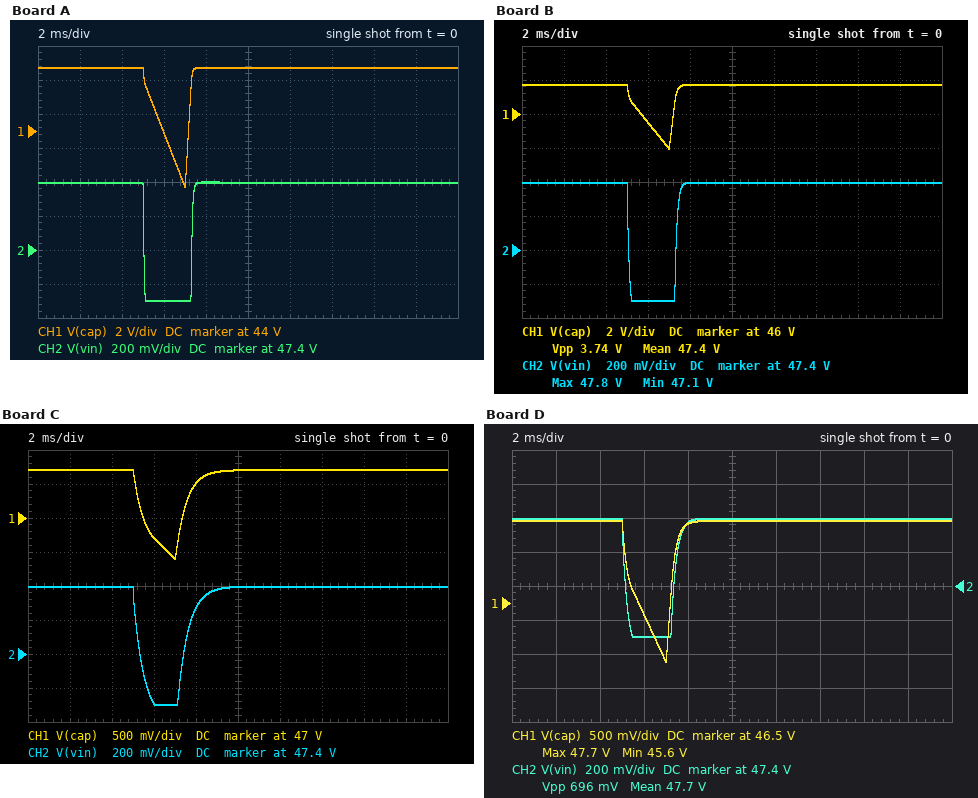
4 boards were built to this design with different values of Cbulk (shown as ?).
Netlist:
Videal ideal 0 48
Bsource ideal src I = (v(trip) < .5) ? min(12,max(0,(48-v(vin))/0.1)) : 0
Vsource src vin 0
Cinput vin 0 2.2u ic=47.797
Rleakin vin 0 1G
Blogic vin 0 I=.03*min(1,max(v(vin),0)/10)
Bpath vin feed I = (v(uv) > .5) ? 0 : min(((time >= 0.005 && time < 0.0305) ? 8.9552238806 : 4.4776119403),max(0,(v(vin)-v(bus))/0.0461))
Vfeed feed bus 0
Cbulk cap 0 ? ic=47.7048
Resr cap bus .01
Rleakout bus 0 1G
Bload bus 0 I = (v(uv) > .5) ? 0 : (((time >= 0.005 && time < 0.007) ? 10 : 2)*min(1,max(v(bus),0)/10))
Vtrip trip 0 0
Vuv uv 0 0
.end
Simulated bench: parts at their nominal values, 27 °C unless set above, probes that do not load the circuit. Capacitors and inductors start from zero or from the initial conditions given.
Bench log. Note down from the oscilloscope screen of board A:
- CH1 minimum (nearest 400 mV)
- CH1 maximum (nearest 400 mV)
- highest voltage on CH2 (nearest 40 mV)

40.8 V
47.6 V
47.80 V
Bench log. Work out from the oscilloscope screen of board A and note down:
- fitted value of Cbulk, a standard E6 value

330 µF
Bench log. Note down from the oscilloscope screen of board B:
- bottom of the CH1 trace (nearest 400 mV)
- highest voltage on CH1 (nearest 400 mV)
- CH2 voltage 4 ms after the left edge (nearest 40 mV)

44.0 V
47.6 V
47.80 V
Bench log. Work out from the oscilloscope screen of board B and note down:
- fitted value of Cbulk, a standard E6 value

680 µF
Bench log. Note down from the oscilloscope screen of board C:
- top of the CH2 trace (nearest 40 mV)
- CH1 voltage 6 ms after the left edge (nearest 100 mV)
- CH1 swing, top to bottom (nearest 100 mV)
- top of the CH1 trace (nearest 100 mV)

47.80 V
46.7 V
1.3 V
47.7 V
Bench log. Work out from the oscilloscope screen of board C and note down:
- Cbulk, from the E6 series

3.3 mF
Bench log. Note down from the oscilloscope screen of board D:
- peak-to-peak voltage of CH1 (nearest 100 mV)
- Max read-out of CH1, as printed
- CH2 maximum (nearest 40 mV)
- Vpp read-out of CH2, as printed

2.1 V
47.7 V
47.80 V
696 mV
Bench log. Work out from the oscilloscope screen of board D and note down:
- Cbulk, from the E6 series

1.5 mF
